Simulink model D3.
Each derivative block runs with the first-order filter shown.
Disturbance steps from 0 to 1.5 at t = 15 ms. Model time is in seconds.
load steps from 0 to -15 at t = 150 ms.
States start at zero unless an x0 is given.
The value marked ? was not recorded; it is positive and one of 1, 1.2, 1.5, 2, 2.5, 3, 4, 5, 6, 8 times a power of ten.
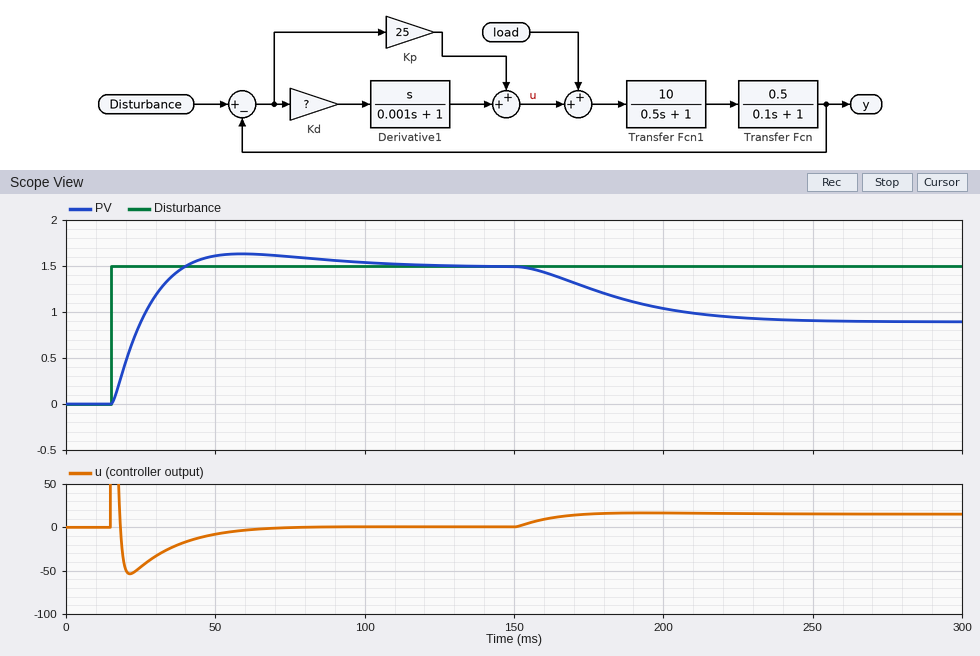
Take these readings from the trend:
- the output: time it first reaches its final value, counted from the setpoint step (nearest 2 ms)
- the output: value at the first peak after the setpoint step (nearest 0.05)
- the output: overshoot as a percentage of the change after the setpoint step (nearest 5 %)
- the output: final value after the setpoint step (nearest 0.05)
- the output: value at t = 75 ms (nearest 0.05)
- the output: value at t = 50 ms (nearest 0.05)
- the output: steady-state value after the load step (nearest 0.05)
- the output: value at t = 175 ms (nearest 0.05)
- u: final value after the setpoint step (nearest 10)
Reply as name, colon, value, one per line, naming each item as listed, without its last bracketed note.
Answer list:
the output: time it first reaches its final value, counted from the setpoint step: 24 ms
the output: value at the first peak after the setpoint step: 1.65
the output: overshoot as a percentage of the change after the setpoint step: 10 %
the output: final value after the setpoint step: 1.50
the output: value at t = 75 ms: 1.60
the output: value at t = 50 ms: 1.60
the output: steady-state value after the load step: 0.90
the output: value at t = 175 ms: 1.25
u: final value after the setpoint step: 0
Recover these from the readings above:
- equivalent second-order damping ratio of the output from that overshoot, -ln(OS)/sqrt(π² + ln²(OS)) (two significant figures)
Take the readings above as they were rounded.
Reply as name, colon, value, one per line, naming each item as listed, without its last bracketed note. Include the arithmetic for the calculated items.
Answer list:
equivalent second-order damping ratio of the output from that overshoot, -ln(OS)/sqrt(π² + ln²(OS)): ln(0.1) = -2.303; 2.303 / sqrt(9.870 + 5.302) = 0.59
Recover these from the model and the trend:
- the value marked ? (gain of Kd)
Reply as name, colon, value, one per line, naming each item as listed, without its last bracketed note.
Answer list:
the value marked ?: 0.8
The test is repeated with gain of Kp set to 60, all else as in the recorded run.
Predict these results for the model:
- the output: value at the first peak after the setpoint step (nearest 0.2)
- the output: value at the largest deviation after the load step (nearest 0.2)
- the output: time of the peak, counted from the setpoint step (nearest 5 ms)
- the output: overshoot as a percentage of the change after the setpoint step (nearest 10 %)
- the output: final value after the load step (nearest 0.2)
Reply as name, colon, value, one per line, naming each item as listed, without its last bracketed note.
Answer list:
the output: value at the first peak after the setpoint step: 1.8
the output: value at the largest deviation after the load step: 1.2
the output: time of the peak, counted from the setpoint step: 30 ms
the output: overshoot as a percentage of the change after the setpoint step: 20 %
the output: final value after the load step: 1.2
